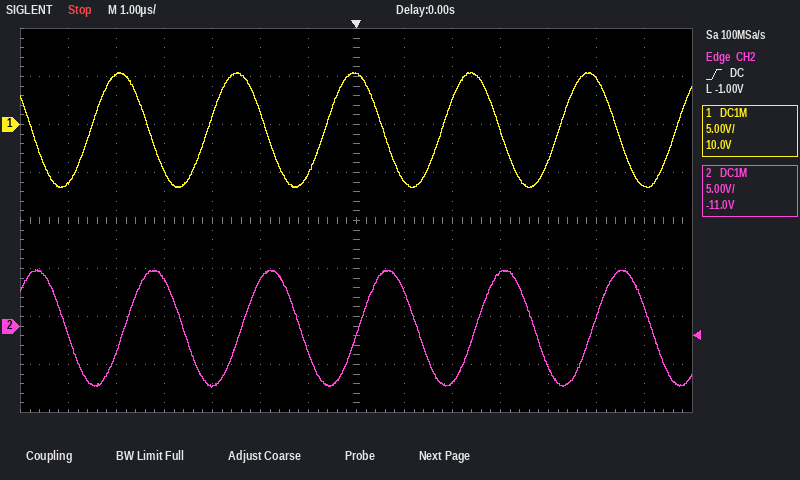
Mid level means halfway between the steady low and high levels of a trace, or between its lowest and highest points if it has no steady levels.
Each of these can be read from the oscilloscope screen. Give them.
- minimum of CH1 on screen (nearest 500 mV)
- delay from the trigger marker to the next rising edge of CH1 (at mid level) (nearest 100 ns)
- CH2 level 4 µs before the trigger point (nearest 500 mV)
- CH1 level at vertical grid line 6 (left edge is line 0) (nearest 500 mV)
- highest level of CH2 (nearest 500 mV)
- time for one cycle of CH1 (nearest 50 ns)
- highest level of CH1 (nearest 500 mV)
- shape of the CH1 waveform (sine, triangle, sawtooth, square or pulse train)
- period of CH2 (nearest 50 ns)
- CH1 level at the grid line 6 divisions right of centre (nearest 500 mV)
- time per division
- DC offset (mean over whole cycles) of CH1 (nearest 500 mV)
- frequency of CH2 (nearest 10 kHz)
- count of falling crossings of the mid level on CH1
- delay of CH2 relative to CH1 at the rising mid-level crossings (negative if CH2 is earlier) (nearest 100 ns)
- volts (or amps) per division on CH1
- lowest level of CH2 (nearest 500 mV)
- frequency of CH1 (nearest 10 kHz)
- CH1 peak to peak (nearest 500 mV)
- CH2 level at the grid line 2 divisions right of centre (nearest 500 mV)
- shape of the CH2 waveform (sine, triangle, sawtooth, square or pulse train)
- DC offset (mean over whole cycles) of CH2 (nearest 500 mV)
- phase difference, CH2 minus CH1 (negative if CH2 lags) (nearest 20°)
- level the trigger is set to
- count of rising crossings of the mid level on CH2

-6.5 V
1.8 µs
5.0 V
-5.0 V
6.0 V
2.45 µs
5.5 V
sine
2.45 µs
-6.5 V
1 µs
-500 mV
410 kHz
6
+700 ns
5 V
-6.5 V
410 kHz
12.0 V
-6.0 V
sine
0.0 V
-100°
-1.00 V
5
